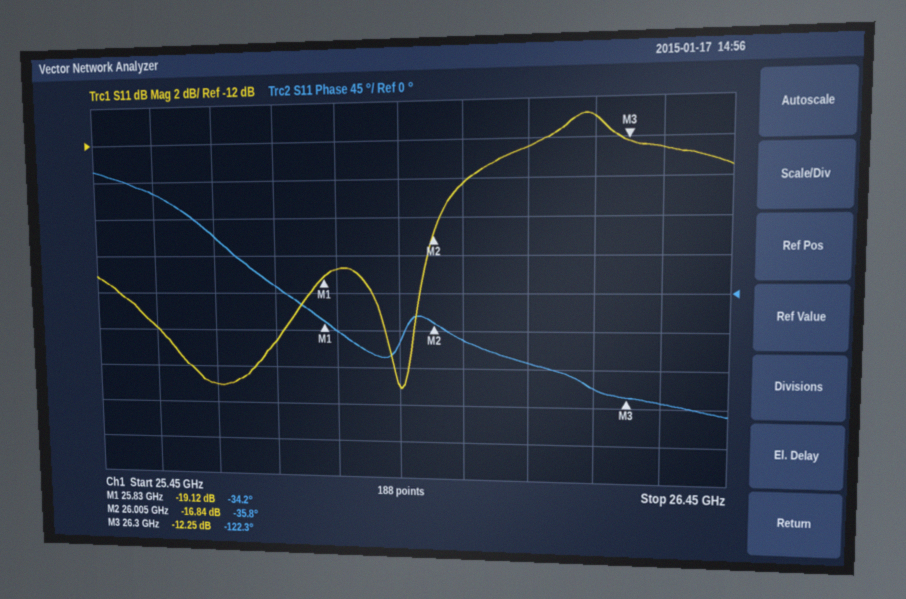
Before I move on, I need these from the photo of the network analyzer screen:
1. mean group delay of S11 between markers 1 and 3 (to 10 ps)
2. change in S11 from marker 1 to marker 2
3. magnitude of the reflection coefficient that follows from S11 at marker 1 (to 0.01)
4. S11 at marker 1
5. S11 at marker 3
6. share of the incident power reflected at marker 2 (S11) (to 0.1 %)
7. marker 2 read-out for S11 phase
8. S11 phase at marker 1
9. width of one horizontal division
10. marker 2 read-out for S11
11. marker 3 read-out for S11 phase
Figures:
520 ps
2.28 dB
0.11
-19.12 dB
-12.25 dB
2.1 %
-35.8°
-34.2°
100 MHz
-16.84 dB
-122.3°
